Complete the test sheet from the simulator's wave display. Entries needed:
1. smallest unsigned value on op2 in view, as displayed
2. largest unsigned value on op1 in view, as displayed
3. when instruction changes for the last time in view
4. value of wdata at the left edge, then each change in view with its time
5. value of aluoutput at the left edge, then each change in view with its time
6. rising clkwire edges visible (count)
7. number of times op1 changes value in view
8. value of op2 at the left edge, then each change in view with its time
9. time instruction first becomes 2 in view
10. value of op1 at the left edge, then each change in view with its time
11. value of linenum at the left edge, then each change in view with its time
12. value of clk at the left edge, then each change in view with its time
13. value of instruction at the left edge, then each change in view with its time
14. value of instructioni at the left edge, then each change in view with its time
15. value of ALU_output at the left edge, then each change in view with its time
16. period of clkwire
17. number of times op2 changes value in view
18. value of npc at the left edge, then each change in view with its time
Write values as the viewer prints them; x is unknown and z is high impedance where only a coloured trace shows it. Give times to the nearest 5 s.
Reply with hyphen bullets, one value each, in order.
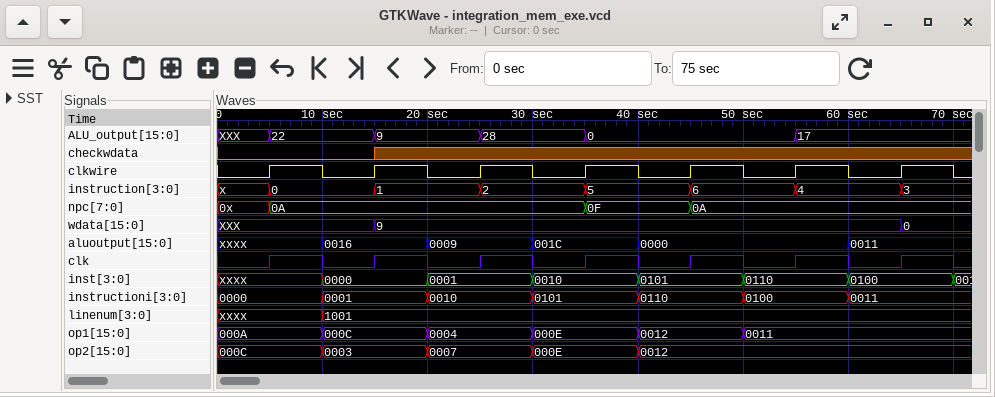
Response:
- 0003
- 0012
- 65 s
- XXX, 9 at 15 s, 0 at 65 s
- xxxx, 0016 at 10 s, 0009 at 20 s, 001C at 30 s, 0000 at 40 s, 0011 at 60 s
- 7
- 5
- 000C, 0003 at 10 s, 0007 at 20 s, 000E at 30 s, 0012 at 40 s
- 25 s
- 000A, 000C at 10 s, 0004 at 20 s, 000E at 30 s, 0012 at 40 s, 0011 at 50 s
- xxxx, 1001 at 10 s
- 0, 1 at 5 s, 0 at 10 s, 1 at 15 s, 0 at 20 s, 1 at 25 s, 0 at 30 s, 1 at 35 s, 0 at 40 s, 1 at 45 s, 0 at 50 s, 1 at 55 s, 0 at 60 s, 1 at 65 s, 0 at 70 s
- x, 0 at 5 s, 1 at 15 s, 2 at 25 s, 5 at 35 s, 6 at 45 s, 4 at 55 s, 3 at 65 s
- 0000, 0001 at 10 s, 0010 at 20 s, 0101 at 30 s, 0110 at 40 s, 0100 at 50 s, 0011 at 60 s
- XXX, 22 at 5 s, 9 at 15 s, 28 at 25 s, 0 at 35 s, 17 at 55 s
- 10 s
- 4
- 0x, 0A at 5 s, 0F at 35 s, 0A at 45 s
